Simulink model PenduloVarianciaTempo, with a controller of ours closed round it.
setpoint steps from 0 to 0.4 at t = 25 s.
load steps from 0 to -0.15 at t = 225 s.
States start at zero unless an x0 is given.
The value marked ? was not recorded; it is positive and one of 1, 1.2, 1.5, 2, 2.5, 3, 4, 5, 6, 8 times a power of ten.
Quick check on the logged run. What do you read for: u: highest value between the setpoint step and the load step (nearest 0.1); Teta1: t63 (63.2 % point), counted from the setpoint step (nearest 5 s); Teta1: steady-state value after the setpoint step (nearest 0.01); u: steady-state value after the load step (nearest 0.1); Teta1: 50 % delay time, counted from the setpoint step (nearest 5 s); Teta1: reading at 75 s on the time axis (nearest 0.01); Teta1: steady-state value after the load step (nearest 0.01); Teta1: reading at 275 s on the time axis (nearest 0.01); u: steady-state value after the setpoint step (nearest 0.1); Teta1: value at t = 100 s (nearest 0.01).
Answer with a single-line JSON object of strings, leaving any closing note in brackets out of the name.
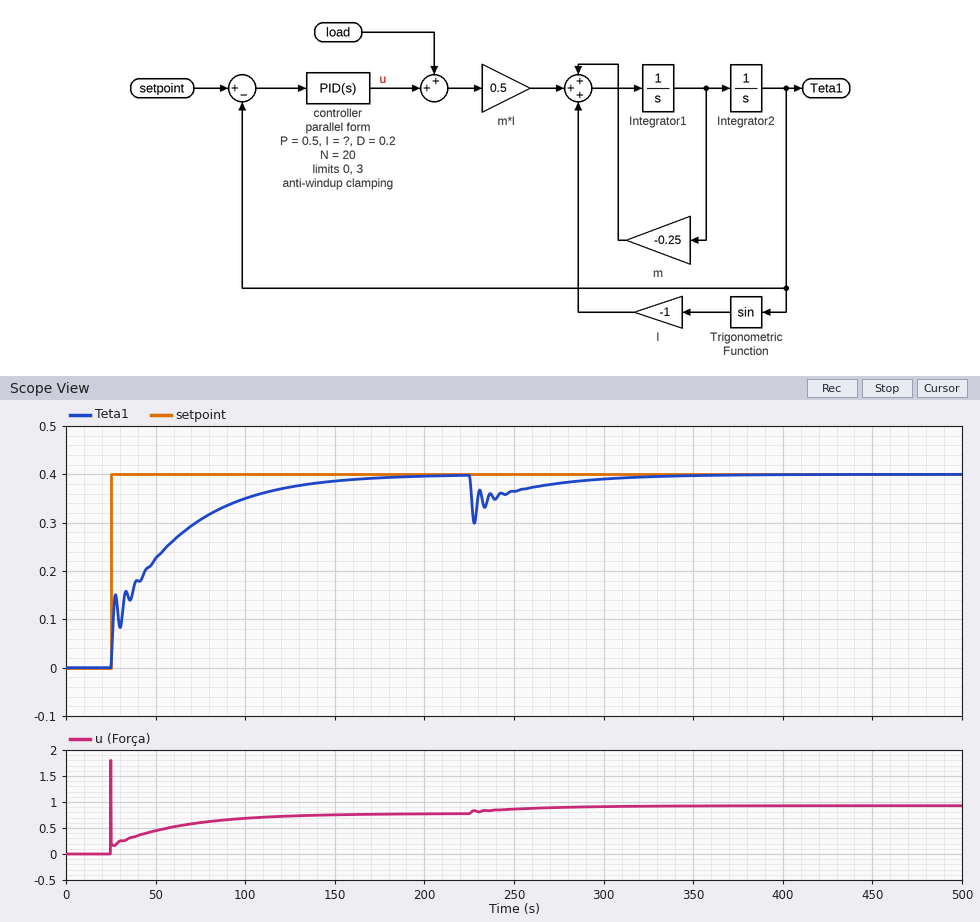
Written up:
{"u: highest value between the setpoint step and the load step": "1.8", "Teta1: t63 (63.2 % point), counted from the setpoint step": "30 s", "Teta1: steady-state value after the setpoint step": "0.40", "u: steady-state value after the load step": "0.9", "Teta1: 50 % delay time, counted from the setpoint step": "20 s", "Teta1: reading at 75 s on the time axis": "0.31", "Teta1: steady-state value after the load step": "0.40", "Teta1: reading at 275 s on the time axis": "0.38", "u: steady-state value after the setpoint step": "0.8", "Teta1: value at t = 100 s": "0.35"}
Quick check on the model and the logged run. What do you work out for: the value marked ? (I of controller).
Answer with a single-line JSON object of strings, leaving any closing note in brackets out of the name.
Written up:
{"the value marked ?": "0.06"}
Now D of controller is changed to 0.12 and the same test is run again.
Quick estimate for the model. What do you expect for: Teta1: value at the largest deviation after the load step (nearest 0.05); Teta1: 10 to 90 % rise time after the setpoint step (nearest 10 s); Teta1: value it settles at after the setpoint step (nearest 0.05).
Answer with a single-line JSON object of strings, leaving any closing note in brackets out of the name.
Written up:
{"Teta1: value at the largest deviation after the load step": "0.30", "Teta1: 10 to 90 % rise time after the setpoint step": "80 s", "Teta1: value it settles at after the setpoint step": "0.40"}
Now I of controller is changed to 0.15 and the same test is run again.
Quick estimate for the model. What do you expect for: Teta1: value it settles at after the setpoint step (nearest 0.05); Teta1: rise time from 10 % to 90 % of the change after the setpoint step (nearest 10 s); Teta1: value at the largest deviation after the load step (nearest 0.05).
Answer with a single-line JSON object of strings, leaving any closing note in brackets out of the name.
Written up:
{"Teta1: value it settles at after the setpoint step": "0.40", "Teta1: rise time from 10 % to 90 % of the change after the setpoint step": "30 s", "Teta1: value at the largest deviation after the load step": "0.30"}
